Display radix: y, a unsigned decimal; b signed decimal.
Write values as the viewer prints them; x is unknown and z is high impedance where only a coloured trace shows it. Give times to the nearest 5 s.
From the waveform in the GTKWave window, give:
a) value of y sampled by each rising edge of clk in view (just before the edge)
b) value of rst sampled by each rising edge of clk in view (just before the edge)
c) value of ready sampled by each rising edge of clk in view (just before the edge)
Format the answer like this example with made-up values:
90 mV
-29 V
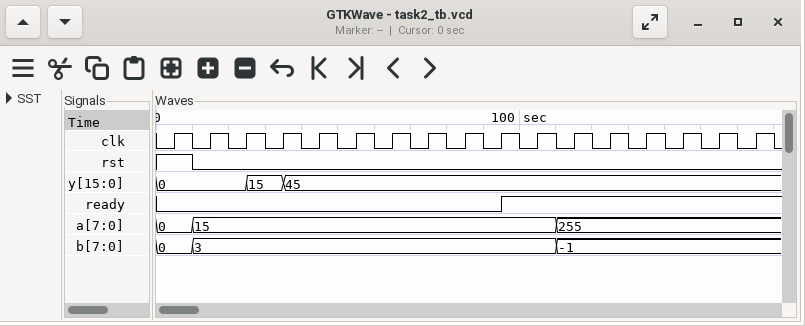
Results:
0, 0, 0, 15, 45, 45, 45, 45, 45, 45, 45, 45, 45, 45, 45, 45, 45
1 0 0 0 0 0 0 0 0 0 0 0 0 0 0 0 0
0 0 0 0 0 0 0 0 0 0 1 1 1 1 1 1 1
